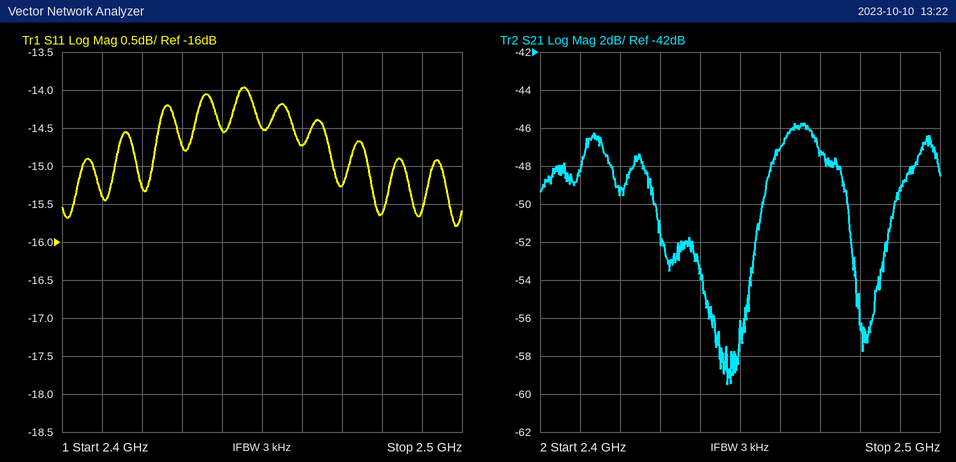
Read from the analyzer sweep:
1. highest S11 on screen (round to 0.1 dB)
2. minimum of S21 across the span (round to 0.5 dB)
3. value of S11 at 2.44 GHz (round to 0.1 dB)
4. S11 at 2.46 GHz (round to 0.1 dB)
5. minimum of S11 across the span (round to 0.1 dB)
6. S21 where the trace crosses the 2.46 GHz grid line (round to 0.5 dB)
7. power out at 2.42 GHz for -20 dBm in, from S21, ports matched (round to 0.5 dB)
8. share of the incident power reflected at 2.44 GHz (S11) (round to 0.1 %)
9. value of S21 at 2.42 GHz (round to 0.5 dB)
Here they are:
-14.0 dB
-59.5 dB
-14.5 dB
-14.7 dB
-15.8 dB
-47.0 dB
-69.5 dBm
3.5 %
-49.5 dB
